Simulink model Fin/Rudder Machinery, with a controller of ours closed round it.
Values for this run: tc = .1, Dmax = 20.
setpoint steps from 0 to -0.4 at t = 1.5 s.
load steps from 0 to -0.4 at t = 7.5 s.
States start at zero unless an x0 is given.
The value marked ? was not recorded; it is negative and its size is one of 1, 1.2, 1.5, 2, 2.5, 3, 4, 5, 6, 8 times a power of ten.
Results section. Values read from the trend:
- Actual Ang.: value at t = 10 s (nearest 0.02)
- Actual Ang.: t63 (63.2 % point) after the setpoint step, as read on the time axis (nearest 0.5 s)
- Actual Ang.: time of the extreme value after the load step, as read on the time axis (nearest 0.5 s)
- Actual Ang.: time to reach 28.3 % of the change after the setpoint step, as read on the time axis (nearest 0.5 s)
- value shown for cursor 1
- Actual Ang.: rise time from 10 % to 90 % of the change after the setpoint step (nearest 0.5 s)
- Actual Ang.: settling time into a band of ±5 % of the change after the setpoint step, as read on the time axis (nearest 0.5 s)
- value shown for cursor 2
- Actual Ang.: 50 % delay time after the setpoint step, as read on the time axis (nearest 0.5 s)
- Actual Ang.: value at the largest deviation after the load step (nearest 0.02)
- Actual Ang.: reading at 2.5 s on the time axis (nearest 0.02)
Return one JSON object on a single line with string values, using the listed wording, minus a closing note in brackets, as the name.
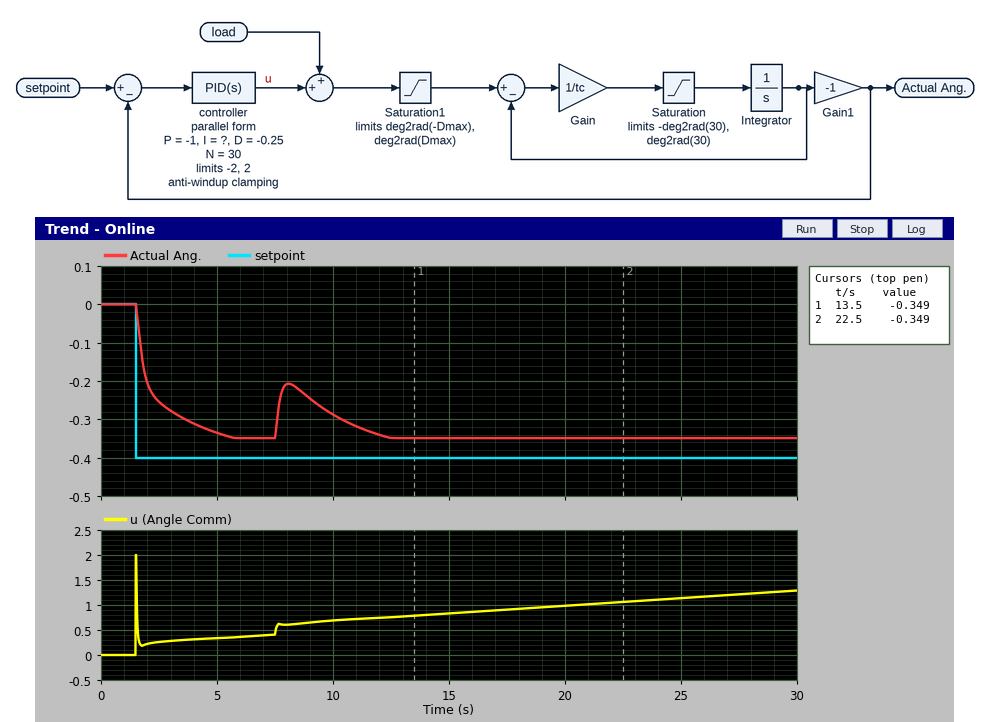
{"Actual Ang.: value at t = 10 s": "-0.28", "Actual Ang.: t63 (63.2 % point) after the setpoint step, as read on the time axis": "2.0 s", "Actual Ang.: time of the extreme value after the load step, as read on the time axis": "8.0 s", "Actual Ang.: time to reach 28.3 % of the change after the setpoint step, as read on the time axis": "1.5 s", "value shown for cursor 1": "-0.349", "Actual Ang.: rise time from 10 % to 90 % of the change after the setpoint step": "2.5 s", "Actual Ang.: settling time into a band of ±5 % of the change after the setpoint step, as read on the time axis": "5.0 s", "value shown for cursor 2": "-0.349", "Actual Ang.: 50 % delay time after the setpoint step, as read on the time axis": "2.0 s", "Actual Ang.: value at the largest deviation after the load step": "-0.20", "Actual Ang.: reading at 2.5 s on the time axis": "-0.26"}
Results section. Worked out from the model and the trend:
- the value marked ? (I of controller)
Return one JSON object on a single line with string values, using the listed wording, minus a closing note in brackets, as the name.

{"the value marked ?": "-0.6"}
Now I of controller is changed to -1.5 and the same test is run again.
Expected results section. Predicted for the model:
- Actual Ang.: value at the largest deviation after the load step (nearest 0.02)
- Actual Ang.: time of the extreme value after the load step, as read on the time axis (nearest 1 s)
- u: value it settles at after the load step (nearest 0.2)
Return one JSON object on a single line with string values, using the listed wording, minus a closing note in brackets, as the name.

{"Actual Ang.: value at the largest deviation after the load step": "-0.34", "Actual Ang.: time of the extreme value after the load step, as read on the time axis": "8 s", "u: value it settles at after the load step": "2.0"}
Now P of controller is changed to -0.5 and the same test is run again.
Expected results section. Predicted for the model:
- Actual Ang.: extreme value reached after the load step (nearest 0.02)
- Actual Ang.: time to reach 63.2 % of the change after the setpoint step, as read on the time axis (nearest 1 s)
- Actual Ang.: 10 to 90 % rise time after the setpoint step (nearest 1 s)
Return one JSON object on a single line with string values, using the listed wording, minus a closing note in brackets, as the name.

{"Actual Ang.: extreme value reached after the load step": "-0.18", "Actual Ang.: time to reach 63.2 % of the change after the setpoint step, as read on the time axis": "3 s", "Actual Ang.: 10 to 90 % rise time after the setpoint step": "3 s"}
